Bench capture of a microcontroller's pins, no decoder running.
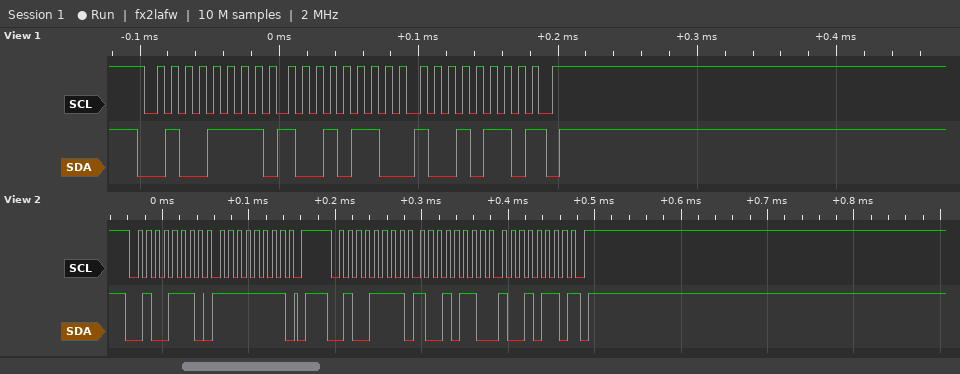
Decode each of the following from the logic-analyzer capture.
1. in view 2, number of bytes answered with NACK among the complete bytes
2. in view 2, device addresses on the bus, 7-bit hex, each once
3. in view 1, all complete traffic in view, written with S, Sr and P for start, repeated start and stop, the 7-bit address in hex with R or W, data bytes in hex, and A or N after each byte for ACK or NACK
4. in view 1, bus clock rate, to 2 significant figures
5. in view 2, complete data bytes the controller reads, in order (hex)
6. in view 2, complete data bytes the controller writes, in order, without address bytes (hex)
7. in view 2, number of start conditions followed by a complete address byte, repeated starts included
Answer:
1
0x27
S 27R A 96 A 96 N P
100 kHz
96 96
FF
2
